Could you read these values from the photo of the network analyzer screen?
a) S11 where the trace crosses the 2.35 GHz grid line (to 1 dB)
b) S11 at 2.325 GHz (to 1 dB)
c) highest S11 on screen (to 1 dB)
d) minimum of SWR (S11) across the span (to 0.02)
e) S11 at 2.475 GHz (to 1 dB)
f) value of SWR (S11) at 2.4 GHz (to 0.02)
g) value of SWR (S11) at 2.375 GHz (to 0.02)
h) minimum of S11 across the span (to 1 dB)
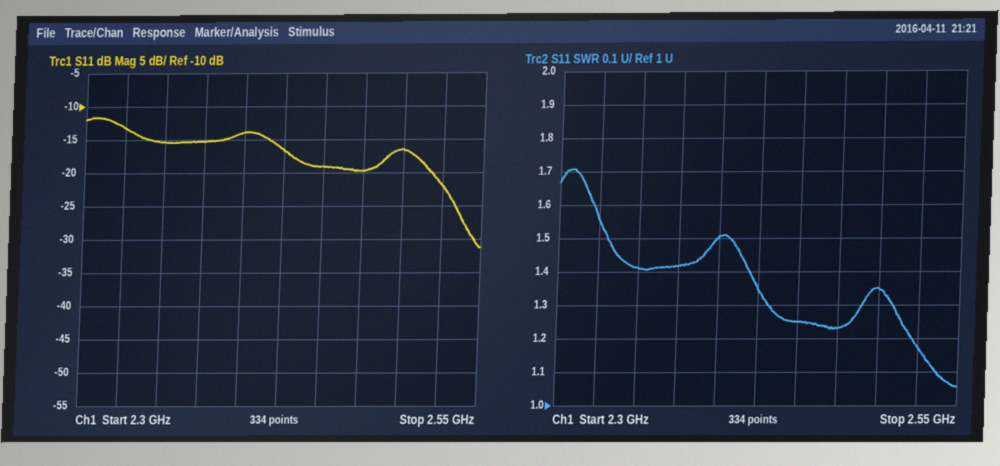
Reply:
-15 dB
-13 dB
-12 dB
1.06
-20 dB
1.50
1.42
-31 dB
